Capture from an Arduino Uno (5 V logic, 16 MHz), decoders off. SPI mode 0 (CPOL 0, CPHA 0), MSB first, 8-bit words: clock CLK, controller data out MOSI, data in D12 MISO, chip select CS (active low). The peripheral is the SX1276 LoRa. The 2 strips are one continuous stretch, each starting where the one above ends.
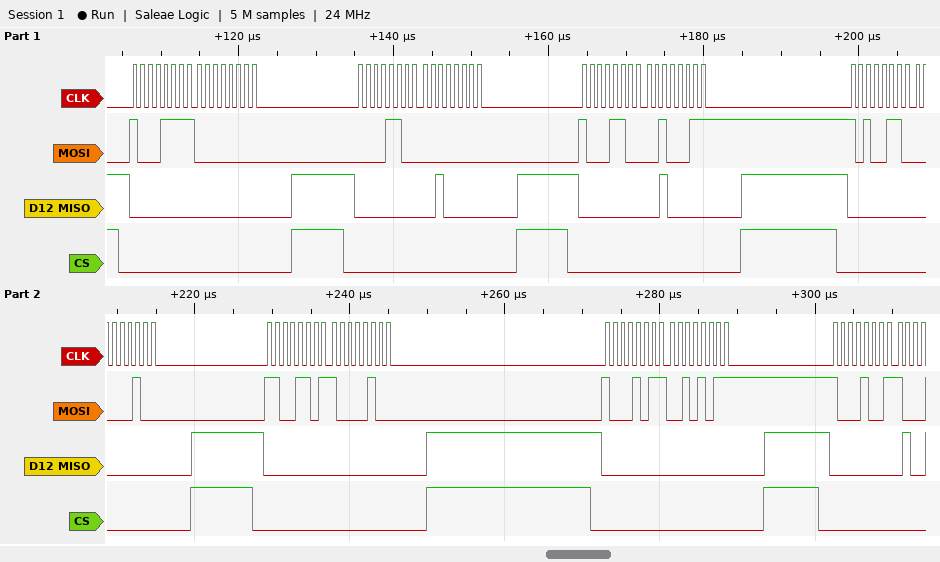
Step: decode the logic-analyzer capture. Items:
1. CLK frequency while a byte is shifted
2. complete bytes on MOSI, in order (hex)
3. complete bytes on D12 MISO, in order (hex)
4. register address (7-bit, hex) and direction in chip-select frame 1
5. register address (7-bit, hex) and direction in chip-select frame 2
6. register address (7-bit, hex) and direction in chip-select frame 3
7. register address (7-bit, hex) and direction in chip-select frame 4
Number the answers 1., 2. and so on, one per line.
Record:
1. 1 MHz
2. 8F 00 0C 00 8C 23 A6 04 CD 84 8B 2B 89
3. 00 00 00 20 00 20 00 00 00 00 00 00 00
4. 0x0F write
5. 0x0C read
6. 0x0C write
7. 0x26 write
